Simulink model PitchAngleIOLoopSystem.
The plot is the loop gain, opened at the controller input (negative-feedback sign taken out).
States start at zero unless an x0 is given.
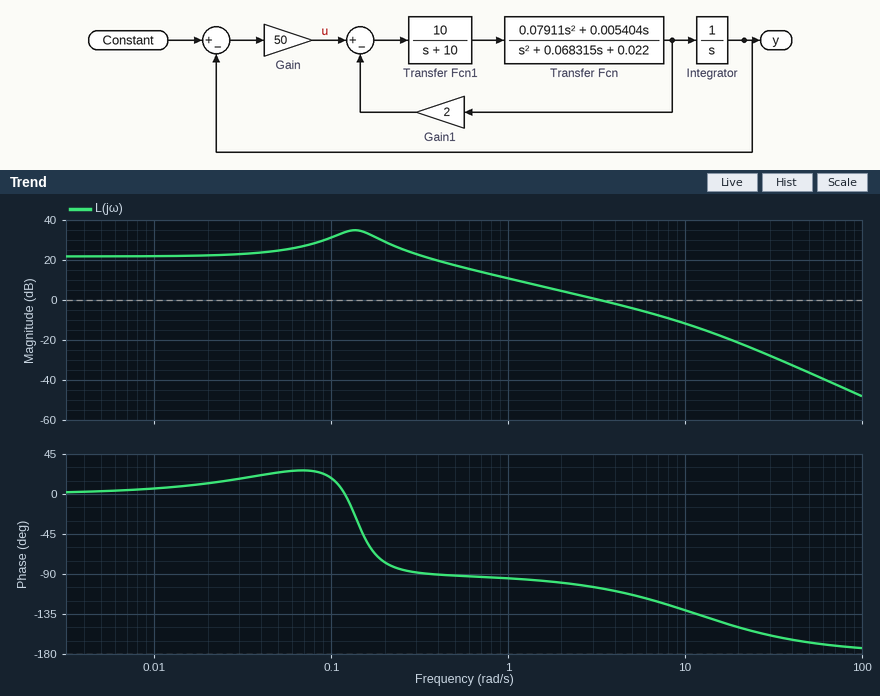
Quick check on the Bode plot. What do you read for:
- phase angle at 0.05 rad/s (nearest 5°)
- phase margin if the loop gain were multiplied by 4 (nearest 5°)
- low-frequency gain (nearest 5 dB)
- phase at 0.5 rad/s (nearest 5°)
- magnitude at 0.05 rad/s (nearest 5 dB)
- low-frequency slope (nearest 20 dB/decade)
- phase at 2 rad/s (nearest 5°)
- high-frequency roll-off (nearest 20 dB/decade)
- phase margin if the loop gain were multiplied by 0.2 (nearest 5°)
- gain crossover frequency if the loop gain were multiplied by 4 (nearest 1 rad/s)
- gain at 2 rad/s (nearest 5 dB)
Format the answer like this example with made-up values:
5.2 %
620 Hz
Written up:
25°
50°
20 dB
-90°
25 dB
0 dB/decade
-100°
-40 dB/decade
85°
10 rad/s
5 dB
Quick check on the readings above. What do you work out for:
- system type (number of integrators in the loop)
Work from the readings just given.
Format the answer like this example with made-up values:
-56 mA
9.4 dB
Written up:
0
